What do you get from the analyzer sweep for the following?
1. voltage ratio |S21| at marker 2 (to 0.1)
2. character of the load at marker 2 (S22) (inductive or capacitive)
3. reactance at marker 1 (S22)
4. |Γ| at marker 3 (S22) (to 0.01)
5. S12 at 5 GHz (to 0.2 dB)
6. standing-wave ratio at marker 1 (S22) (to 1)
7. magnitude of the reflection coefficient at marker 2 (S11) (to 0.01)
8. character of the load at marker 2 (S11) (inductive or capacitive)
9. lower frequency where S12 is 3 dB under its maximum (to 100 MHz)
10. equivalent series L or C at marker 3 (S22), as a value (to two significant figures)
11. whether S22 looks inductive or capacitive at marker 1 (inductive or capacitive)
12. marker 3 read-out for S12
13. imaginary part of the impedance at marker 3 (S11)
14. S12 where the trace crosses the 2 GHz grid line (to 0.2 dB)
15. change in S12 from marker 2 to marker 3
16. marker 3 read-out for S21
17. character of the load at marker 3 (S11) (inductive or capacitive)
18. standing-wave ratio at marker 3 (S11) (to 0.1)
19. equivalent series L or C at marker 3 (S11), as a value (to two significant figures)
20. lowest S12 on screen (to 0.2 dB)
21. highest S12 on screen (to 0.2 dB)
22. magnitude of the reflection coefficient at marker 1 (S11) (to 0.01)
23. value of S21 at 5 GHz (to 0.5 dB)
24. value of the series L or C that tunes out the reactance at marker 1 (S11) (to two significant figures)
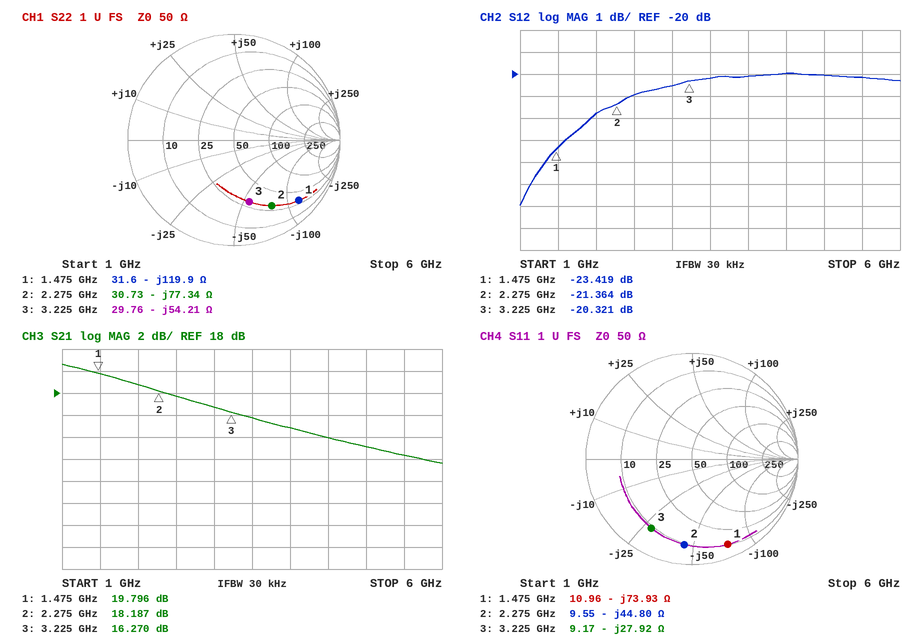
8.1
capacitive
-119.9 Ω
0.60
-20.0 dB
11
0.81
capacitive
1.6 GHz
910 fF
capacitive
-20.321 dB
-27.92 Ω
-21.8 dB
1.043 dB
16.270 dB
capacitive
7.2
1.8 pF
-26.0 dB
-20.0 dB
0.87
13.0 dB
8.0 nH
